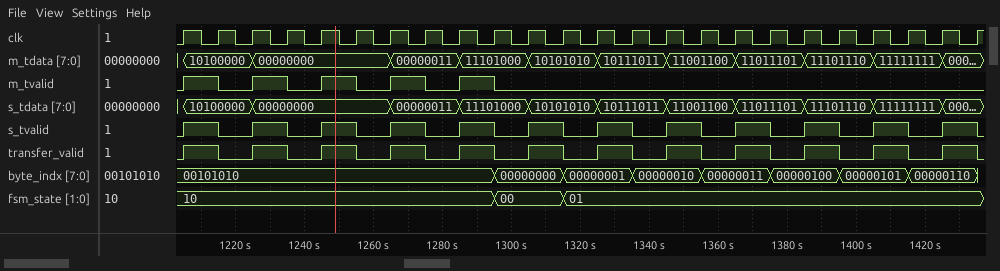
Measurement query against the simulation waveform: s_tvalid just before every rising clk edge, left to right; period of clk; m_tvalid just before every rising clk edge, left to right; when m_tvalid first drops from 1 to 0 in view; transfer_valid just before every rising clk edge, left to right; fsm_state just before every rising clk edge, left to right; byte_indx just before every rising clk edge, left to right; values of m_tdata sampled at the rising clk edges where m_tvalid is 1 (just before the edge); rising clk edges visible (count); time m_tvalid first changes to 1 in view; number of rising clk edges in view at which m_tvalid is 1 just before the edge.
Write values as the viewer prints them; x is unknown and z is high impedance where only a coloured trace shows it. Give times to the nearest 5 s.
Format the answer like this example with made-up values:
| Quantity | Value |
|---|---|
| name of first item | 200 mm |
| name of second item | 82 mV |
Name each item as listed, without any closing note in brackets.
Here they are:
| Quantity | Value |
|---|---|
| s_tvalid just before every rising clk edge, left to right | 0 1 0 1 0 1 0 1 0 1 0 1 0 1 0 1 0 1 0 1 0 1 0 1 |
| period of clk | 10 s |
| m_tvalid just before every rising clk edge, left to right | 0 1 0 1 0 1 0 1 0 1 0 0 0 0 0 0 0 0 0 0 0 0 0 0 |
| when m_tvalid first drops from 1 to 0 in view | 1215 s |
| transfer_valid just before every rising clk edge, left to right | 0 1 0 1 0 1 0 1 0 1 0 1 0 1 0 1 0 1 0 1 0 1 0 1 |
| fsm_state just before every rising clk edge, left to right | 10, 10, 10, 10, 10, 10, 10, 10, 10, 10, 00, 00, 01, 01, 01, 01, 01, 01, 01, 01, 01, 01, 01, 01 |
| byte_indx just before every rising clk edge, left to right | 00101010, 00101010, 00101010, 00101010, 00101010, 00101010, 00101010, 00101010, 00101010, 00101010, 00000000, 00000000, 00000001, 00000001, 00000010, 00000010, 00000011, 00000011, 00000100, 00000100, 00000101, 00000101, 00000110, 00000110 |
| values of m_tdata sampled at the rising clk edges where m_tvalid is 1 | 10100000, 00000000, 00000000, 00000011, 11101000 |
| rising clk edges visible | 24 |
| time m_tvalid first changes to 1 in view | 1205 s |
| number of rising clk edges in view at which m_tvalid is 1 just before the edge | 5 |
